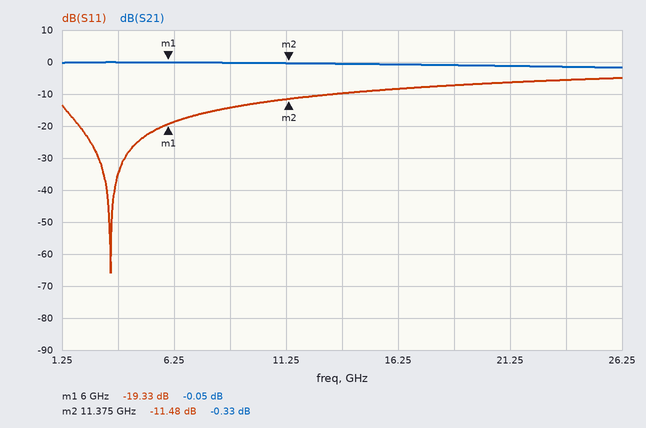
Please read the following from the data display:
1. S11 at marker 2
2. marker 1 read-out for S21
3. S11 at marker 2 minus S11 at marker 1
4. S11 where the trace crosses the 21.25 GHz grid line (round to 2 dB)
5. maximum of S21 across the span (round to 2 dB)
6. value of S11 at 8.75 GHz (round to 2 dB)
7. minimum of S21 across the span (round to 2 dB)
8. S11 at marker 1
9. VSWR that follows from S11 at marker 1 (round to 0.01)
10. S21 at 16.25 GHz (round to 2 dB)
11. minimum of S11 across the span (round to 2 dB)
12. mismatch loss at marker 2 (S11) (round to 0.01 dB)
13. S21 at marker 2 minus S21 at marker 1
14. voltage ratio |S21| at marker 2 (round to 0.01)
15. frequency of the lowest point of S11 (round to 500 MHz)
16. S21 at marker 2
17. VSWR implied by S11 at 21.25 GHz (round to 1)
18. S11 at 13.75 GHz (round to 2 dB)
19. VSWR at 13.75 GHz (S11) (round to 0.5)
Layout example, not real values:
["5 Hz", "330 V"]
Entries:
["-11.48 dB", "-0.05 dB", "7.85 dB", "-6 dB", "0 dB", "-14 dB", "-2 dB", "-19.33 dB", "1.24", "0 dB", "-66 dB", "0.32 dB", "-0.28 dB", "0.96", "3.5 GHz", "-0.33 dB", "3", "-10 dB", "2.0"]
